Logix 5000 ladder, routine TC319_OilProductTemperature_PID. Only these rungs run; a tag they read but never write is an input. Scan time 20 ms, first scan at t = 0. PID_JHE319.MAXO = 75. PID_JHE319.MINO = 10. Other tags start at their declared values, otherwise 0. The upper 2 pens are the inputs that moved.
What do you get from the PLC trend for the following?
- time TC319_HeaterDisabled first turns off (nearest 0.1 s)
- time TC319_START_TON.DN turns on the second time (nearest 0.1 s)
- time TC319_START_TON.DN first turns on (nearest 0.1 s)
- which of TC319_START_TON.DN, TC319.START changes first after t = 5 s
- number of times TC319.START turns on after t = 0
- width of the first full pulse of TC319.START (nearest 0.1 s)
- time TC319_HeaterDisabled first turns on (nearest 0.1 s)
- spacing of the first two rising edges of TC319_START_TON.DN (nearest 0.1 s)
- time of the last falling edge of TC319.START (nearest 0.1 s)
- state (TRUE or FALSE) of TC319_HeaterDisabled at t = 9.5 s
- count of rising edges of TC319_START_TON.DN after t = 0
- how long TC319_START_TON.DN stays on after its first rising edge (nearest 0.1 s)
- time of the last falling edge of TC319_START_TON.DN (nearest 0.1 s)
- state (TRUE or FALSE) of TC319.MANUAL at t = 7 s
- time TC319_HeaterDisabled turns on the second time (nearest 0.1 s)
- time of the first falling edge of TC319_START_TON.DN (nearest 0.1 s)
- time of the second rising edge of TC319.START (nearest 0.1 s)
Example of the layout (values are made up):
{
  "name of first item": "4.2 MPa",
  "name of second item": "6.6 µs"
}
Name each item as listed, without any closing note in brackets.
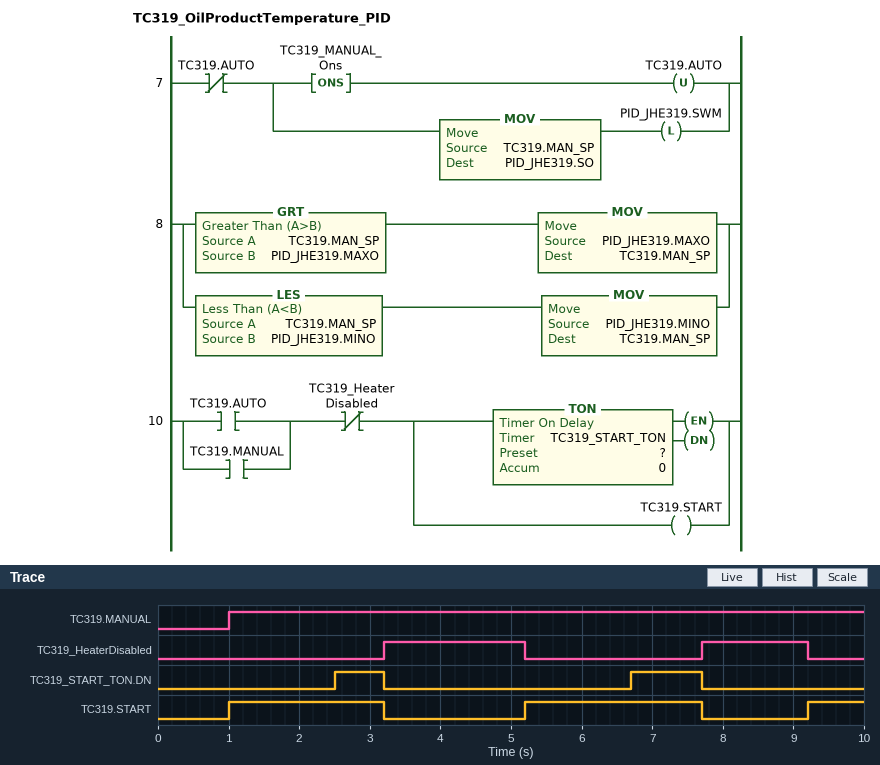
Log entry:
{
  "time TC319_HeaterDisabled first turns off": "5.2 s",
  "time TC319_START_TON.DN turns on the second time": "6.7 s",
  "time TC319_START_TON.DN first turns on": "2.5 s",
  "which of TC319_START_TON.DN, TC319.START changes first after t = 5 s": "TC319.START",
  "number of times TC319.START turns on after t = 0": "3",
  "width of the first full pulse of TC319.START": "2.2 s",
  "time TC319_HeaterDisabled first turns on": "3.2 s",
  "spacing of the first two rising edges of TC319_START_TON.DN": "4.2 s",
  "time of the last falling edge of TC319.START": "7.7 s",
  "state (TRUE or FALSE) of TC319_HeaterDisabled at t = 9.5 s": "FALSE",
  "count of rising edges of TC319_START_TON.DN after t = 0": "2",
  "how long TC319_START_TON.DN stays on after its first rising edge": "0.7 s",
  "time of the last falling edge of TC319_START_TON.DN": "7.7 s",
  "state (TRUE or FALSE) of TC319.MANUAL at t = 7 s": "TRUE",
  "time TC319_HeaterDisabled turns on the second time": "7.7 s",
  "time of the first falling edge of TC319_START_TON.DN": "3.2 s",
  "time of the second rising edge of TC319.START": "5.2 s"
}
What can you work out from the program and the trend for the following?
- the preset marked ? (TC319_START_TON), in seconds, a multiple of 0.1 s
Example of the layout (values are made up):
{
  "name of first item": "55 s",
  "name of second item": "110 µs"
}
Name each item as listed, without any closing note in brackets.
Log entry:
{
  "the preset marked ? (TC319_START_TON), in seconds, a multiple of 0.1 s": "1.5 s"
}
